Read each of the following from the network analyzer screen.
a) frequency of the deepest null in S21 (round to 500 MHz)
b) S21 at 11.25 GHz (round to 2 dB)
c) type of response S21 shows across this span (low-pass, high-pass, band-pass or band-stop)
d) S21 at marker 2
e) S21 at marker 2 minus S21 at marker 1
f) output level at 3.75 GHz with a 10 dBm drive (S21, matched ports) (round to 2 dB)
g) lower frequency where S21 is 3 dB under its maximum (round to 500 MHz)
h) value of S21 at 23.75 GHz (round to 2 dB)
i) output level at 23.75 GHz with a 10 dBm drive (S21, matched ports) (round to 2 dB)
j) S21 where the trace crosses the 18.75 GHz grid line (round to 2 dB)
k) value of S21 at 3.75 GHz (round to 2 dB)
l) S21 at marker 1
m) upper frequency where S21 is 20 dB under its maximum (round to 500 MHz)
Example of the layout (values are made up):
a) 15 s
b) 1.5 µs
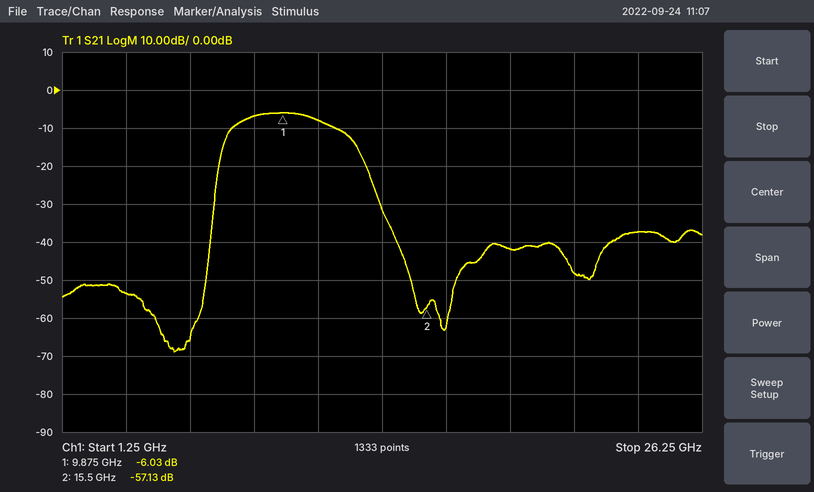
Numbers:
a) 5.5 GHz
b) -8 dB
c) band-pass
d) -57.13 dB
e) -51.10 dB
f) -44 dBm
g) 8.0 GHz
h) -38 dB
i) -28 dBm
j) -42 dB
k) -54 dB
l) -6.03 dB
m) 13.5 GHz
